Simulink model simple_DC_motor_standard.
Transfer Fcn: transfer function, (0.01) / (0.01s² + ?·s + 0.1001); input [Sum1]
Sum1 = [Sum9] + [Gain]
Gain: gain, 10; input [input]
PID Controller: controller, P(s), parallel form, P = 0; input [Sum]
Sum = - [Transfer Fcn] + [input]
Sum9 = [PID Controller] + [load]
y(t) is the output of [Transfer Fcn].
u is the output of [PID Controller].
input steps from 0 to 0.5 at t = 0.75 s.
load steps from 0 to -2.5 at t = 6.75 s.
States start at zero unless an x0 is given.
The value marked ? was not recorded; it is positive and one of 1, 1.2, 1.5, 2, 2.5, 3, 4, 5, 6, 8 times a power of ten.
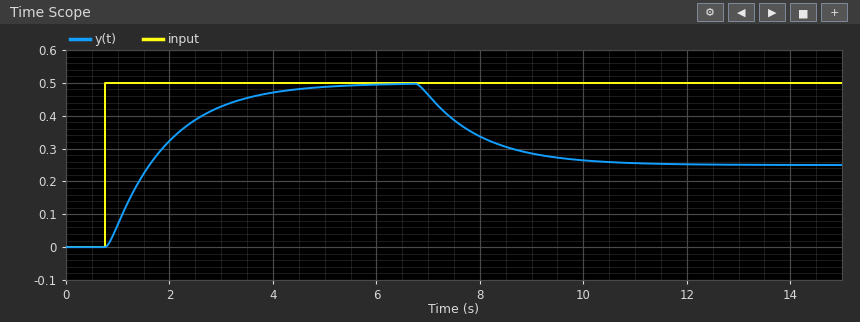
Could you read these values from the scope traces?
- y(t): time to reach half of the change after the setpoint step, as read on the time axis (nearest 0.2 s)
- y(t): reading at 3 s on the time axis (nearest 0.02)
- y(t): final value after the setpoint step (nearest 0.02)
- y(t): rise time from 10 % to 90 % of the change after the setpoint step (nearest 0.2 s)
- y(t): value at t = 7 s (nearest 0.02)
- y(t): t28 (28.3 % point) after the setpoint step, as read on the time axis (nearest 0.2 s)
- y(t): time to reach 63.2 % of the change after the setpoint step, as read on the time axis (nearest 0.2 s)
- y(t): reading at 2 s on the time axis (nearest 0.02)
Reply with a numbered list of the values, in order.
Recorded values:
1. 1.6 s
2. 0.42
3. 0.50
4. 2.4 s
5. 0.46
6. 1.2 s
7. 2.0 s
8. 0.32
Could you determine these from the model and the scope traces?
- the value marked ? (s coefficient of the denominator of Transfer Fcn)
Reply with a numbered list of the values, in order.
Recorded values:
1. 0.12
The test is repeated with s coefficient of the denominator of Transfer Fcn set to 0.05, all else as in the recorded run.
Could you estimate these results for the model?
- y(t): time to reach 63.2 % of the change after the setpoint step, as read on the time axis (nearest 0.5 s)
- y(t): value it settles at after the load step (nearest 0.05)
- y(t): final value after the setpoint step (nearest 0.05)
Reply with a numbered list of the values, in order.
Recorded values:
1. 1.5 s
2. 0.25
3. 0.50
